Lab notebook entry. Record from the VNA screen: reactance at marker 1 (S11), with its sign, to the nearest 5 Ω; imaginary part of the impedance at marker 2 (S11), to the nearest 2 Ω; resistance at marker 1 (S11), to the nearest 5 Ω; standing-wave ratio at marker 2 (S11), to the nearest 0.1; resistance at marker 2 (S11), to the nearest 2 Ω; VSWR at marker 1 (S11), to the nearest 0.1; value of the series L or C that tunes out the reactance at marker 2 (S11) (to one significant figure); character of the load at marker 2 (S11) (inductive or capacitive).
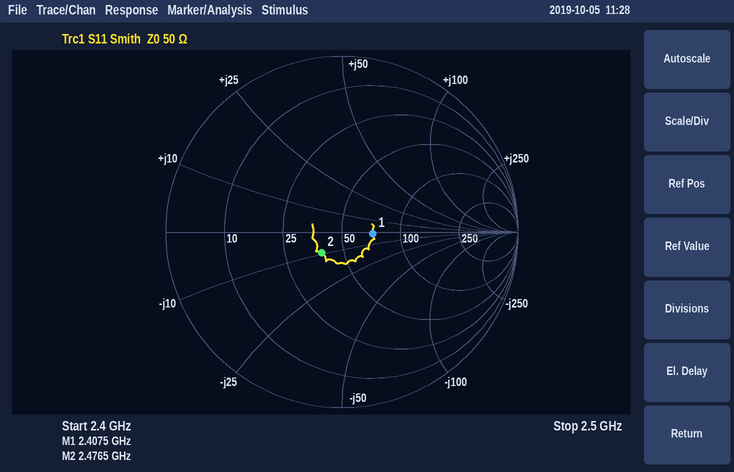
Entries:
0 Ω
-10 Ω
70 Ω
1.4
38 Ω
1.4
600 pH
capacitive
